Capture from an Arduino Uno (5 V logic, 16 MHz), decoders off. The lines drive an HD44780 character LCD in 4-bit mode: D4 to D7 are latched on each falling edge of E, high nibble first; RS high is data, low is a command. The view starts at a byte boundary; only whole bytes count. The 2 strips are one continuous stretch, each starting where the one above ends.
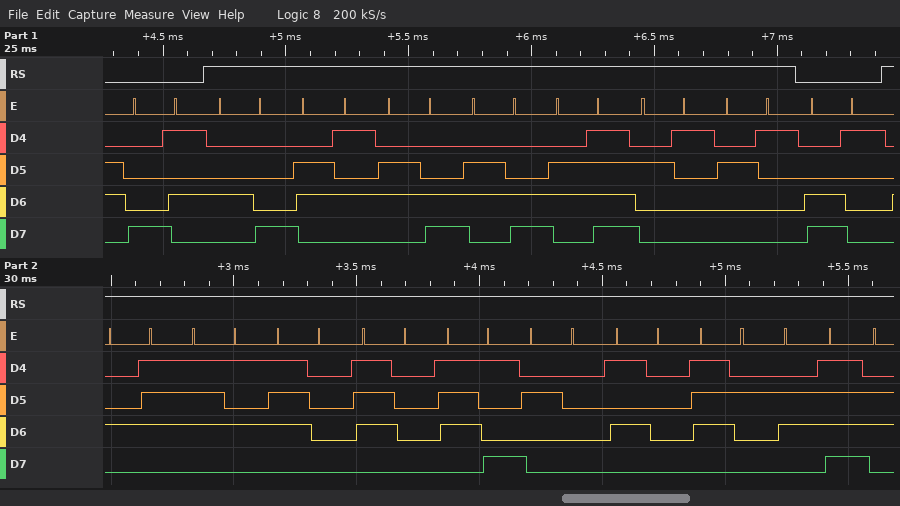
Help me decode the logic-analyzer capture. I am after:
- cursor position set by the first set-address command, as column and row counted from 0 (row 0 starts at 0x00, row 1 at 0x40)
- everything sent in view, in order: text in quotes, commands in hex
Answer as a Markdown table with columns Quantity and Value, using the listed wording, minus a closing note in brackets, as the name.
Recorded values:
| Quantity | Value |
|---|---|
| cursor position set by the first set-address command, as column and row counted from 0 | column 5, row 0 |
| everything sent in view, in order: text in quotes, commands in hex | 0x85 "Hello!!" 0xC1 "Guppy Pro" |
